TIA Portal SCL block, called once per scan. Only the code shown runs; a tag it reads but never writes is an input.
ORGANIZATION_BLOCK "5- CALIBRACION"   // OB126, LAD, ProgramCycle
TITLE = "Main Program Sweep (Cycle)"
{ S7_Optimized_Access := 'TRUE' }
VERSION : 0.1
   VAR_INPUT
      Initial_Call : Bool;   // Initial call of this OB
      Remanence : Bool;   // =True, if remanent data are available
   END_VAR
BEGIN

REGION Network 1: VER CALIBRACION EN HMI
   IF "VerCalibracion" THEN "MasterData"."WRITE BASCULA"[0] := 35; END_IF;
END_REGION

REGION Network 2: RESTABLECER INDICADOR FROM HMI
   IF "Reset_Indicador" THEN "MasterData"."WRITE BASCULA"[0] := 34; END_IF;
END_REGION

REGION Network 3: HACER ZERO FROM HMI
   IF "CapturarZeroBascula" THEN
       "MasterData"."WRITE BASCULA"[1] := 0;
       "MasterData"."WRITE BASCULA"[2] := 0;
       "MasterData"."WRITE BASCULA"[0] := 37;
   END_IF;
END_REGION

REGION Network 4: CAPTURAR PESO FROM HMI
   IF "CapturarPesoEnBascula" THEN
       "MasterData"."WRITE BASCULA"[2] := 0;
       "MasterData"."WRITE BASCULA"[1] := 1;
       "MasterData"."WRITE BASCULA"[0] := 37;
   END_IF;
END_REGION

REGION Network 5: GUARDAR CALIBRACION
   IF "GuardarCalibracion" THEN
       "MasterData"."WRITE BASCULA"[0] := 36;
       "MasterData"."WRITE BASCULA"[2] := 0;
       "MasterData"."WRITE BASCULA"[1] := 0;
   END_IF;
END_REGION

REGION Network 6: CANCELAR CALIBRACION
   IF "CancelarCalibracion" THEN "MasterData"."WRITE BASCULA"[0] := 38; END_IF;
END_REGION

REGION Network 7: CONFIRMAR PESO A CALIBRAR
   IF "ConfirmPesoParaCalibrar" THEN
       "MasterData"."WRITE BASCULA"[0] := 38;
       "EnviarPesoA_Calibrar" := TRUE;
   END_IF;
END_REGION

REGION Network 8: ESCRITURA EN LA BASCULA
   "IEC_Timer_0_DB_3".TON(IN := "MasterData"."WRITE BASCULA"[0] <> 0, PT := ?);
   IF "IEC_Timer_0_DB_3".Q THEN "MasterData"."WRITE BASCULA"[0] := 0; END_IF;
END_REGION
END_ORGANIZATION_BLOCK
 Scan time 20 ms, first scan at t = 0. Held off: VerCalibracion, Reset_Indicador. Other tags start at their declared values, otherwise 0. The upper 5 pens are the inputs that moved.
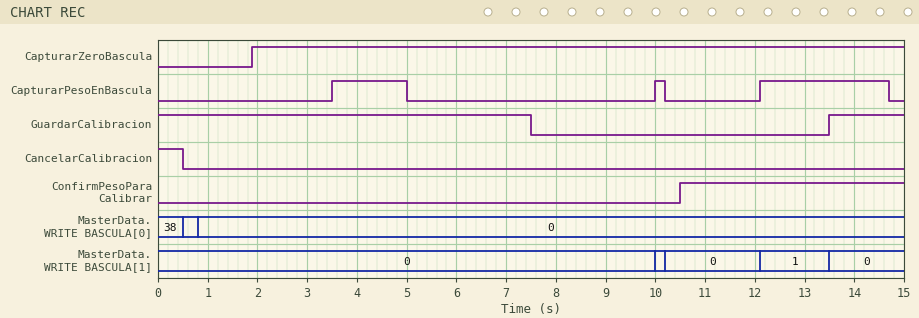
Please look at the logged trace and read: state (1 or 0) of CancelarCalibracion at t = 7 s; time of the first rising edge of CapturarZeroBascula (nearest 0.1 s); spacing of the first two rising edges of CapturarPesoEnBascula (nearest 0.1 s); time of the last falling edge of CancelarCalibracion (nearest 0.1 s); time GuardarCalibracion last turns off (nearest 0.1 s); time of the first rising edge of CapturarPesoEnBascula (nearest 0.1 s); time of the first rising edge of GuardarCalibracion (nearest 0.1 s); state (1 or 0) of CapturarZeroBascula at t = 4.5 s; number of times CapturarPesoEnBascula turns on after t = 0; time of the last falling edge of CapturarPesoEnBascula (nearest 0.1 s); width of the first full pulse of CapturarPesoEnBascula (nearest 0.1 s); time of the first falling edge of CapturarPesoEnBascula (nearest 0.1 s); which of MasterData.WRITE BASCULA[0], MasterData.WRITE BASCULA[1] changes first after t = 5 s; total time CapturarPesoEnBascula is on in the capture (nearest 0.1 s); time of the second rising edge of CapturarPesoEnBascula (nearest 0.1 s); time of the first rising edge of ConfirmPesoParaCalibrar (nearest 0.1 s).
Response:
0
1.9 s
6.5 s
0.5 s
7.5 s
3.5 s
13.5 s
1
3
14.7 s
1.5 s
5.0 s
MasterData.WRITE BASCULA[1]
4.3 s
10.0 s
10.5 s
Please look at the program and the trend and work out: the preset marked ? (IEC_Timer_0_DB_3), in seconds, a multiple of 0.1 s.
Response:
0.8 s
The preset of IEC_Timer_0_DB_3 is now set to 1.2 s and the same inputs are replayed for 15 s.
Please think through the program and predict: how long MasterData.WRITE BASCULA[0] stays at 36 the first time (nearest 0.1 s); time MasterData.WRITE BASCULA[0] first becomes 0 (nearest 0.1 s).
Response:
0.7 s
1.2 s
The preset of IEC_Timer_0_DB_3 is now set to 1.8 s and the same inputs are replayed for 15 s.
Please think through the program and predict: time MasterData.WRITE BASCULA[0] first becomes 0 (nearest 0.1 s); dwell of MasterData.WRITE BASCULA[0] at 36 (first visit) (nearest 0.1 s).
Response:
1.8 s
1.3 s
